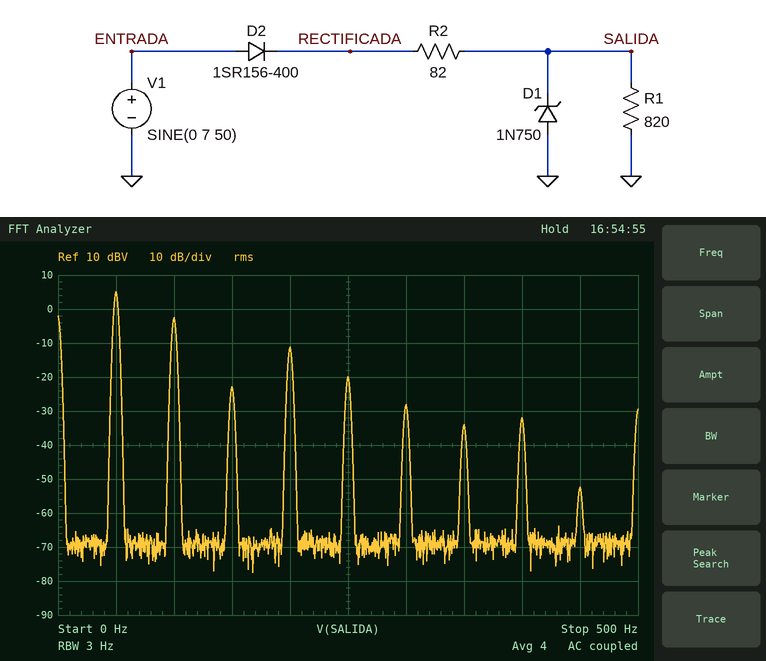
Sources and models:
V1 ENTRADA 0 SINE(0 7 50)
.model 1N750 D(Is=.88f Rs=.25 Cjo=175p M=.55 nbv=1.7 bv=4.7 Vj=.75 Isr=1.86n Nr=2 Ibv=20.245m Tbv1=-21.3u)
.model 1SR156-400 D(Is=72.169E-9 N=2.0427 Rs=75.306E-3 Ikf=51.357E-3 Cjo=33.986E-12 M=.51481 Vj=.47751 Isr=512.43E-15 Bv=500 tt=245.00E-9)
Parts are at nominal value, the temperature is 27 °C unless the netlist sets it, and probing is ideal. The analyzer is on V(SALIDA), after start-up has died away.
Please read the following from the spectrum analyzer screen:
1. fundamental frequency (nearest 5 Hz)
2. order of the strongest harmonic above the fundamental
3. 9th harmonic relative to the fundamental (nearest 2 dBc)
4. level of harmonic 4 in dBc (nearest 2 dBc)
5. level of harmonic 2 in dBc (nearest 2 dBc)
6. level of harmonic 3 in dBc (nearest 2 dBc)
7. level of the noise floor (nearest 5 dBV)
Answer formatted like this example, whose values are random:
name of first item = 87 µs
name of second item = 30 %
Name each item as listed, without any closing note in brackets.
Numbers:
fundamental frequency = 50 Hz
order of the strongest harmonic above the fundamental = 2
9th harmonic relative to the fundamental = -58 dBc
level of harmonic 4 in dBc = -16 dBc
level of harmonic 2 in dBc = -8 dBc
level of harmonic 3 in dBc = -28 dBc
level of the noise floor = -70 dBV
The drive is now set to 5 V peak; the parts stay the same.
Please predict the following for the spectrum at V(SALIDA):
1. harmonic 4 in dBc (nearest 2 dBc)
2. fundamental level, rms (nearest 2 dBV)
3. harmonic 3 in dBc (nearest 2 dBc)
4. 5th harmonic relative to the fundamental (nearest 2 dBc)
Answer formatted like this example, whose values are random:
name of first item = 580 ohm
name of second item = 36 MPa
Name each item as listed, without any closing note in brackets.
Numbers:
harmonic 4 in dBc = -22 dBc
fundamental level, rms = 2 dBV
harmonic 3 in dBc = -26 dBc
5th harmonic relative to the fundamental = -32 dBc
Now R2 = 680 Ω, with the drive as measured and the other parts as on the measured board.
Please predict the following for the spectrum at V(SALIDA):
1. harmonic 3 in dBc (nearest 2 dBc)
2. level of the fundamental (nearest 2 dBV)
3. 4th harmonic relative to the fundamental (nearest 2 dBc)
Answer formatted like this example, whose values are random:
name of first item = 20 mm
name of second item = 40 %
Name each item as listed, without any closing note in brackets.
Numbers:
harmonic 3 in dBc = -30 dBc
level of the fundamental = 2 dBV
4th harmonic relative to the fundamental = -22 dBc
